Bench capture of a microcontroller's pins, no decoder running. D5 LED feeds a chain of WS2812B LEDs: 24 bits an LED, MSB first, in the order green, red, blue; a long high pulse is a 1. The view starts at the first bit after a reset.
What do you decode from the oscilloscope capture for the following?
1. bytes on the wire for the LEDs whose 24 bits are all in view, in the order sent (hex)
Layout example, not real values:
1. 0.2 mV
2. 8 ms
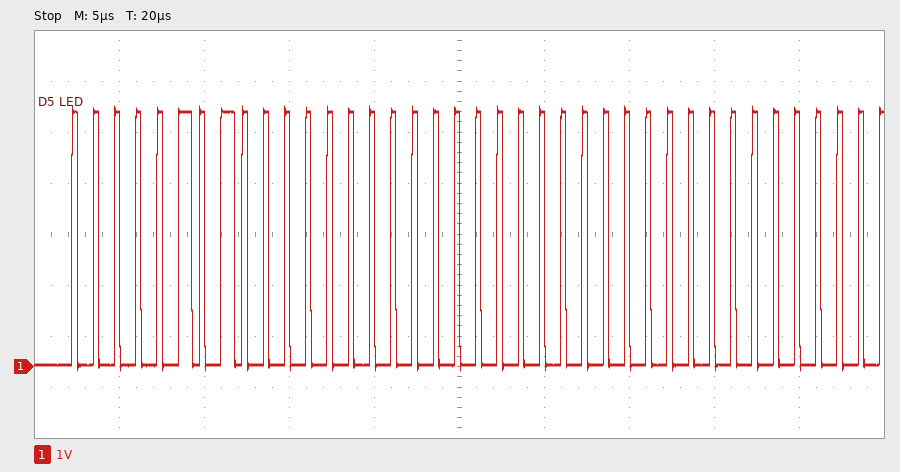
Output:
1. 05 00 00
